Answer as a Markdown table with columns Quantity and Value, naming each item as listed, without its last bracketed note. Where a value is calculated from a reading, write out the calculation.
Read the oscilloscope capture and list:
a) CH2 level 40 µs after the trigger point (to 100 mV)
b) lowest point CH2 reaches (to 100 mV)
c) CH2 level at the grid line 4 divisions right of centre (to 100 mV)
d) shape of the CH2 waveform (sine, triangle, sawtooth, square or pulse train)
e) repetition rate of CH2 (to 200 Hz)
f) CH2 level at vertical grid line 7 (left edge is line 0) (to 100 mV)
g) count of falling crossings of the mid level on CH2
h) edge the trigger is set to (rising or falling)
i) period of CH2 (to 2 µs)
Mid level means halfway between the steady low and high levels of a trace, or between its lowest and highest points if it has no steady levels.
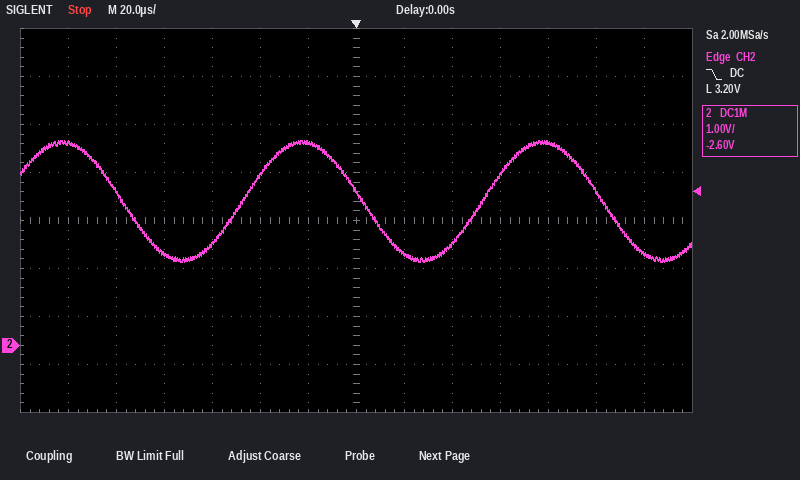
| Quantity | Value |
|---|---|
| CH2 level 40 µs after the trigger point | 2.1 V |
| lowest point CH2 reaches | 1.7 V |
| CH2 level at the grid line 4 divisions right of centre | 4.2 V |
| shape of the CH2 waveform | sine |
| repetition rate of CH2 | 1 / 100 µs ≈ 10.0 kHz |
| CH2 level at vertical grid line 7 (left edge is line 0) | 3.2 V |
| count of falling crossings of the mid level on CH2 | 3 |
| edge the trigger is set to | falling |
| period of CH2 | 100 µs |
